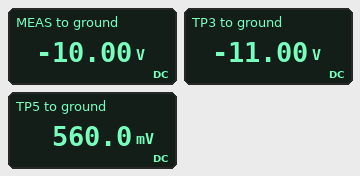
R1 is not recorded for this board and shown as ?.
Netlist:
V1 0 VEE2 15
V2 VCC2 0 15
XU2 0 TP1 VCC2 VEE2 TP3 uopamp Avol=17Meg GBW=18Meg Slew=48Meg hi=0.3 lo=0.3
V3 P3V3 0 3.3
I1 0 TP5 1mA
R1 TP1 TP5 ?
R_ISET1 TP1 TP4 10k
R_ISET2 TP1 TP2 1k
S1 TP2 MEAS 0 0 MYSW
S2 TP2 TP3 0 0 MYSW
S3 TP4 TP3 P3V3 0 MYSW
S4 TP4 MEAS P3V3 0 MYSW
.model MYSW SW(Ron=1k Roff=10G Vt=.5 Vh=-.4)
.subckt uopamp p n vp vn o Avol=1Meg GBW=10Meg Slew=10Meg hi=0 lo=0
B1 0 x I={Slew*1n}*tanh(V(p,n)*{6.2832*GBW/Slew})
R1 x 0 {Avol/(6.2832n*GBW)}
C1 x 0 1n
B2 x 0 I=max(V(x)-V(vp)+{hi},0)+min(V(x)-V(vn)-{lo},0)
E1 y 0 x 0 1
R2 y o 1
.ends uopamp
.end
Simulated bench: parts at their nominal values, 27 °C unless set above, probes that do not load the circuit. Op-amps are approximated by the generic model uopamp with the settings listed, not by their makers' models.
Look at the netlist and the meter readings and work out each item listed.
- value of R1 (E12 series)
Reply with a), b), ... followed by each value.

a) 560 Ω
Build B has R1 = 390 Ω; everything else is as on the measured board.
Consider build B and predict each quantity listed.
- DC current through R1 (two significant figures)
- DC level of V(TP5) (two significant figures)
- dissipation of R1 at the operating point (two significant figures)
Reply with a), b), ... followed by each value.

a) 1.0 mA
b) 390 mV
c) 390 µW
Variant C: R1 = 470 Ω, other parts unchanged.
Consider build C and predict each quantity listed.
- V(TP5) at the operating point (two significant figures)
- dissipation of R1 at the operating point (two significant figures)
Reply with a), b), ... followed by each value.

a) 470 mV
b) 470 µW
